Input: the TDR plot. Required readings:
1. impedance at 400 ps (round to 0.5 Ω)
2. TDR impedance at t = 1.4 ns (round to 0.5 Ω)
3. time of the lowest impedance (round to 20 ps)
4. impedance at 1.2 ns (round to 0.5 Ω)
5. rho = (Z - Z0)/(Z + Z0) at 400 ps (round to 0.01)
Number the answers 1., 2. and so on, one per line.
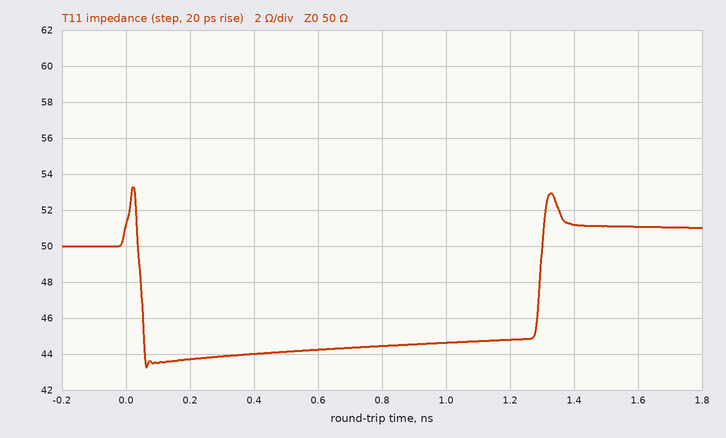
1. 44.0 Ω
2. 51.0 Ω
3. 60 ps
4. 45.0 Ω
5. -0.06
